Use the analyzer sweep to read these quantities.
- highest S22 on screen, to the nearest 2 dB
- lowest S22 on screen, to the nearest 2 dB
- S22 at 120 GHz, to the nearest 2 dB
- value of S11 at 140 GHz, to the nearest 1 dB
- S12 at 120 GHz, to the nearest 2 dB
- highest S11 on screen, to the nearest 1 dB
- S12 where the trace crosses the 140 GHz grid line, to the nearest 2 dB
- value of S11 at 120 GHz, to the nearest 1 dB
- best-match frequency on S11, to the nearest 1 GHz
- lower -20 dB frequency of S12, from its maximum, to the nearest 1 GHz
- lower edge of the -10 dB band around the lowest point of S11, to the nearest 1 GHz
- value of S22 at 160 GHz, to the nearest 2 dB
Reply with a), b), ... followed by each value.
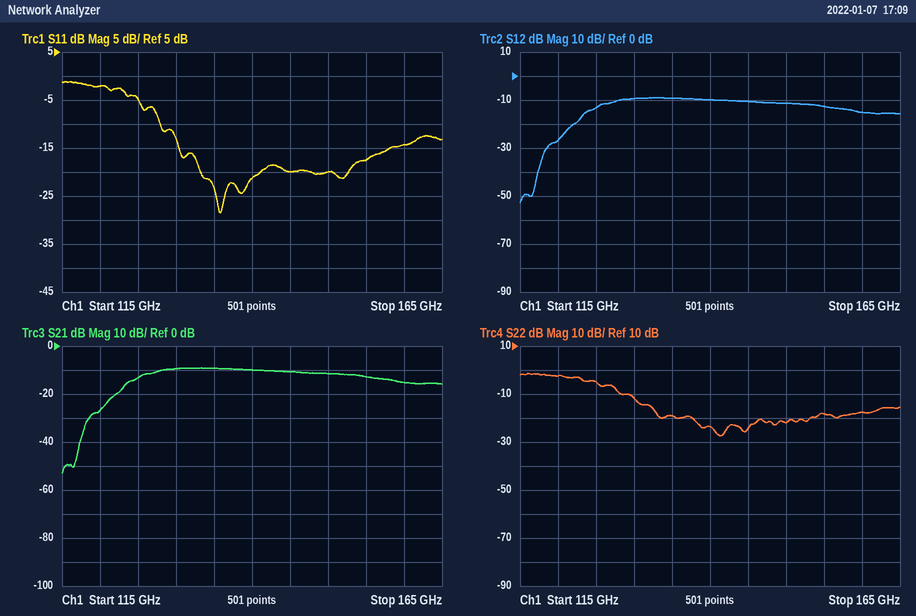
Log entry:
a) -2 dB
b) -28 dB
c) -2 dB
d) -21 dB
e) -26 dB
f) -1 dB
g) -10 dB
h) -2 dB
i) 136 GHz
j) 119 GHz
k) 128 GHz
l) -18 dB
